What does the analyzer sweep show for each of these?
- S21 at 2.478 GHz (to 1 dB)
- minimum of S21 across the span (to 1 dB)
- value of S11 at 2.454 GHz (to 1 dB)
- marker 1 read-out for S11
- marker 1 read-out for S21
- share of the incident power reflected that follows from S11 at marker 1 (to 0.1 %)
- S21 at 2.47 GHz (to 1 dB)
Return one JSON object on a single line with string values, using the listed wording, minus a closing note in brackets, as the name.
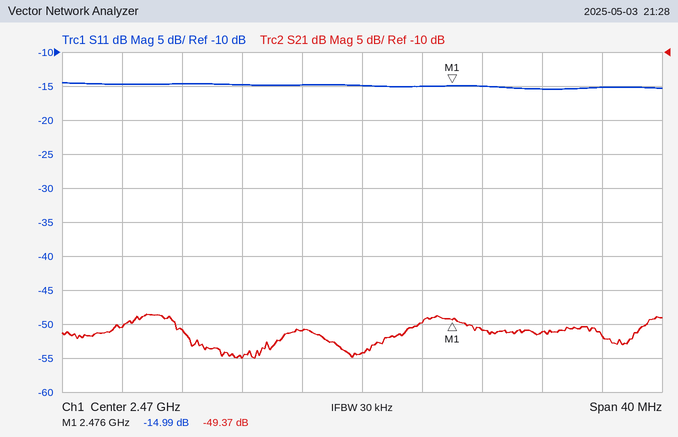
{"S21 at 2.478 GHz": "-51 dB", "minimum of S21 across the span": "-55 dB", "value of S11 at 2.454 GHz": "-15 dB", "marker 1 read-out for S11": "-14.99 dB", "marker 1 read-out for S21": "-49.37 dB", "share of the incident power reflected that follows from S11 at marker 1": "3.2 %", "S21 at 2.47 GHz": "-54 dB"}
